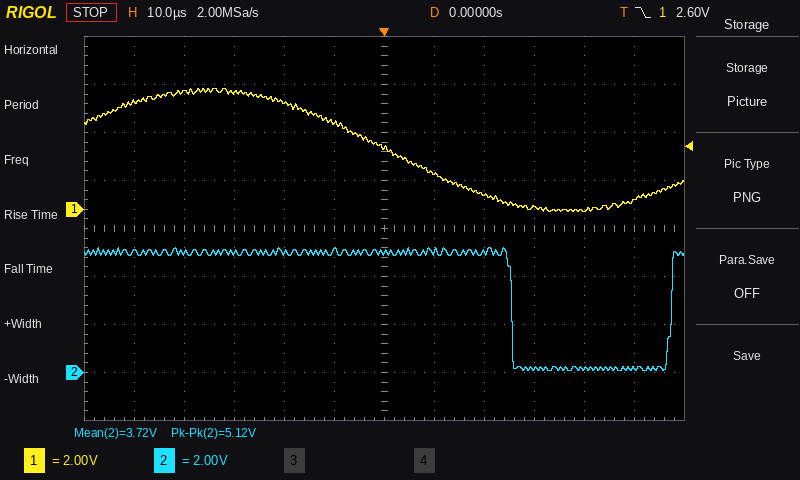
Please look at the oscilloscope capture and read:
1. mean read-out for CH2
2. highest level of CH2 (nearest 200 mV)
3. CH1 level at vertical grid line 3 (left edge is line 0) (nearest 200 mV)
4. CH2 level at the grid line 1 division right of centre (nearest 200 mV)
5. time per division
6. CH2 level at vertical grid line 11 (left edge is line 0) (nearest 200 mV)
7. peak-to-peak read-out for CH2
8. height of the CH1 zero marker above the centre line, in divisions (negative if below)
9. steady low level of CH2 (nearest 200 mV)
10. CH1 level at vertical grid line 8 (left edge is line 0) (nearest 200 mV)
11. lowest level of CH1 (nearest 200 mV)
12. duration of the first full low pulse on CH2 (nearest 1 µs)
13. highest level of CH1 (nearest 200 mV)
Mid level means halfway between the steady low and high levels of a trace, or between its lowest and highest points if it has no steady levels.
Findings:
3.72 V
5.2 V
4.8 V
5.0 V
10 µs
200 mV
5.12 V
+0.4 div
200 mV
600 mV
0.0 V
32 µs
5.0 V
